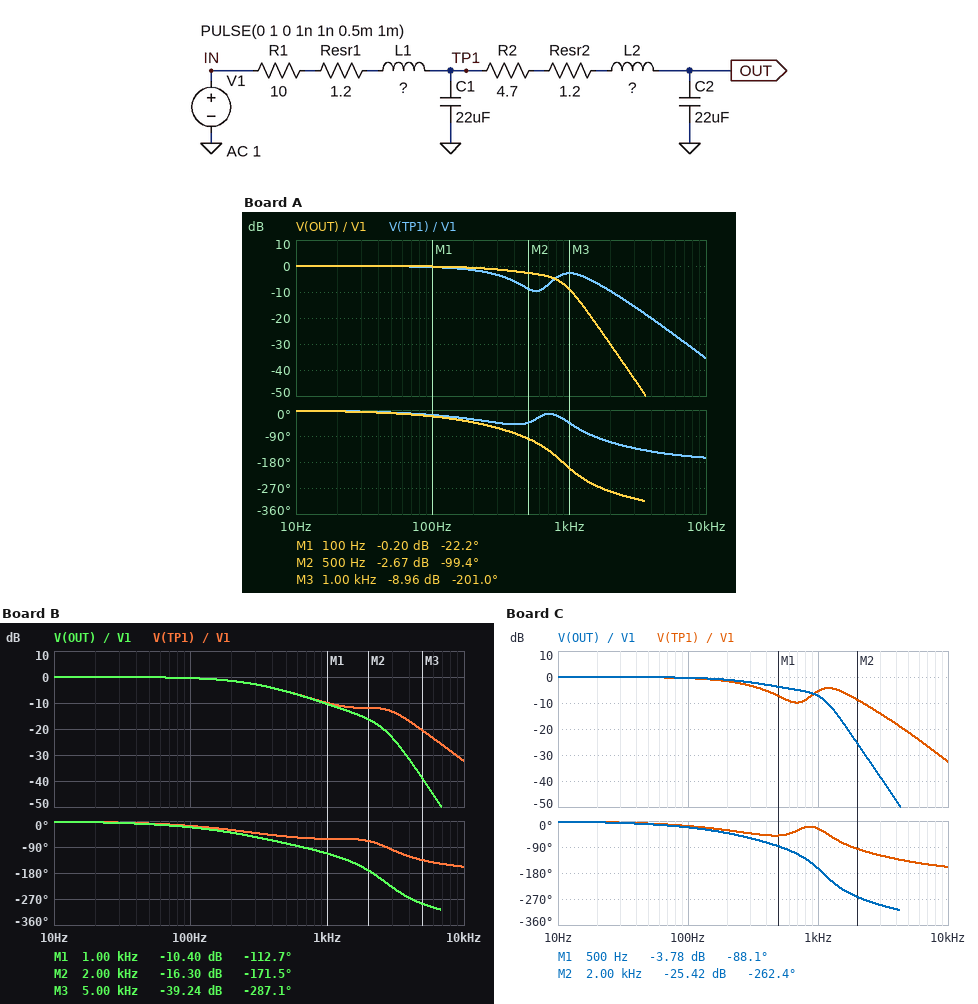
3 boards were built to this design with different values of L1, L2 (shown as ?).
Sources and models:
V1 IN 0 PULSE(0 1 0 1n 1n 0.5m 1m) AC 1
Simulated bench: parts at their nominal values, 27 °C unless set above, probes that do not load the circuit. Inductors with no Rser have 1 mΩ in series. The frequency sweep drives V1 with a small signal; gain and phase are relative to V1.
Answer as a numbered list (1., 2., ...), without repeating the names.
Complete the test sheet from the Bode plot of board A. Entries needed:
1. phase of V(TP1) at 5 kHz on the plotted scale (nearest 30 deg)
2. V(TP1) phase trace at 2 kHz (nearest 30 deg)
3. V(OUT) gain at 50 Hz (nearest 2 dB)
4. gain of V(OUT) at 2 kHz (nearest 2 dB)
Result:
1. -150 deg
2. -120 deg
3. 0 dB
4. -30 dB
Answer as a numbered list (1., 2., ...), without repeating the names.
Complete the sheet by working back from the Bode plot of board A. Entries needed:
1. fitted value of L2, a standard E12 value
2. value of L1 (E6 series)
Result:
1. 3.3 mH
2. 680 µH
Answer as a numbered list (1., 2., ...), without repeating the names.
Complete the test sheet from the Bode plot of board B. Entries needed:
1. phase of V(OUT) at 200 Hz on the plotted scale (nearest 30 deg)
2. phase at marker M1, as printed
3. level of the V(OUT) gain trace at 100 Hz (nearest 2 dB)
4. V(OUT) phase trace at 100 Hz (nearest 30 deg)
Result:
1. -30 deg
2. -112.7 deg
3. 0 dB
4. -30 deg
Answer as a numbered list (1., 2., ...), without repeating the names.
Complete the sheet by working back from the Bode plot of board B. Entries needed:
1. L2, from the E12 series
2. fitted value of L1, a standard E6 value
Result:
1. 390 µH
2. 470 µH
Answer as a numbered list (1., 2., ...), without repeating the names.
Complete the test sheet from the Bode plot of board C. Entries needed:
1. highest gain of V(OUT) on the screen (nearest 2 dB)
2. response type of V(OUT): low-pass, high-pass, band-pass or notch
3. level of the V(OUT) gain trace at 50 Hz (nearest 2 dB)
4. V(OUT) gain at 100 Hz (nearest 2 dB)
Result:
1. 0 dB
2. low-pass
3. 0 dB
4. 0 dB
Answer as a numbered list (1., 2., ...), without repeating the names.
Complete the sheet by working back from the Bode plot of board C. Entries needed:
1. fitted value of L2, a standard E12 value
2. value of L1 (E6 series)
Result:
1. 2.2 mH
2. 470 µH
